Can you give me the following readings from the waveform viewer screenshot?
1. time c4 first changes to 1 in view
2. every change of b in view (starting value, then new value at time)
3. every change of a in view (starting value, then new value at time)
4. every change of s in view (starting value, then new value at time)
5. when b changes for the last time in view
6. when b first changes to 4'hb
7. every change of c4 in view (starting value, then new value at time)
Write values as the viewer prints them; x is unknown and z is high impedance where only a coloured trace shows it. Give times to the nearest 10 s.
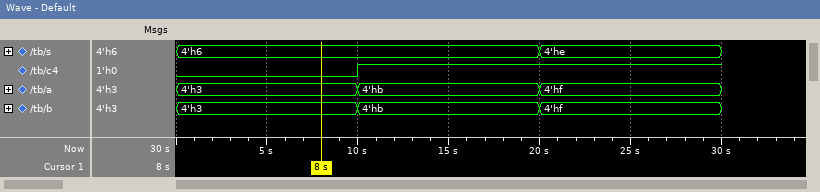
10 s
4'h3, 4'hb at 10 s, 4'hf at 20 s
4'h3, 4'hb at 10 s, 4'hf at 20 s
4'h6, 4'he at 20 s
20 s
10 s
0, 1 at 10 s
